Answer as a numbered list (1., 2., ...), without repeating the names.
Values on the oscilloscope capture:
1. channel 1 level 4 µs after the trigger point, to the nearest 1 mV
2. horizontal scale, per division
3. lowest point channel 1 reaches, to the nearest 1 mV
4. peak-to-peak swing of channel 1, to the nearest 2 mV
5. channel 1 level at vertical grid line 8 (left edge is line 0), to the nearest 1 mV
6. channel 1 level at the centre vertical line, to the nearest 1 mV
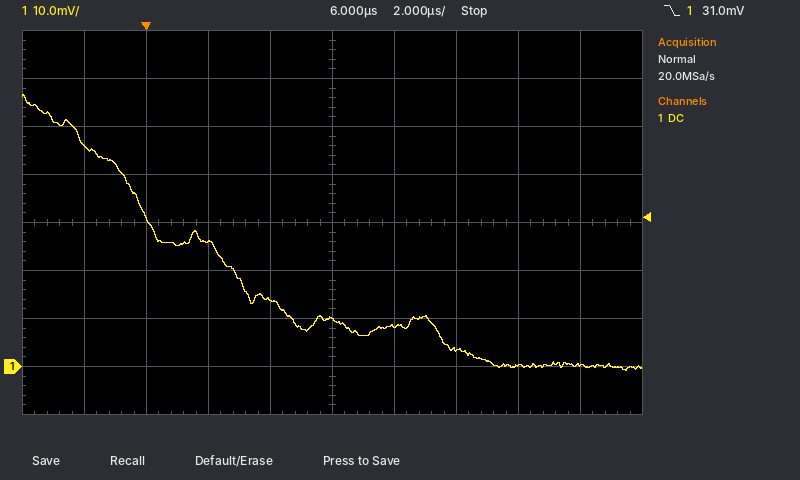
1. 14 mV
2. 2 µs
3. -1 mV
4. 58 mV
5. 0 mV
6. 10 mV
